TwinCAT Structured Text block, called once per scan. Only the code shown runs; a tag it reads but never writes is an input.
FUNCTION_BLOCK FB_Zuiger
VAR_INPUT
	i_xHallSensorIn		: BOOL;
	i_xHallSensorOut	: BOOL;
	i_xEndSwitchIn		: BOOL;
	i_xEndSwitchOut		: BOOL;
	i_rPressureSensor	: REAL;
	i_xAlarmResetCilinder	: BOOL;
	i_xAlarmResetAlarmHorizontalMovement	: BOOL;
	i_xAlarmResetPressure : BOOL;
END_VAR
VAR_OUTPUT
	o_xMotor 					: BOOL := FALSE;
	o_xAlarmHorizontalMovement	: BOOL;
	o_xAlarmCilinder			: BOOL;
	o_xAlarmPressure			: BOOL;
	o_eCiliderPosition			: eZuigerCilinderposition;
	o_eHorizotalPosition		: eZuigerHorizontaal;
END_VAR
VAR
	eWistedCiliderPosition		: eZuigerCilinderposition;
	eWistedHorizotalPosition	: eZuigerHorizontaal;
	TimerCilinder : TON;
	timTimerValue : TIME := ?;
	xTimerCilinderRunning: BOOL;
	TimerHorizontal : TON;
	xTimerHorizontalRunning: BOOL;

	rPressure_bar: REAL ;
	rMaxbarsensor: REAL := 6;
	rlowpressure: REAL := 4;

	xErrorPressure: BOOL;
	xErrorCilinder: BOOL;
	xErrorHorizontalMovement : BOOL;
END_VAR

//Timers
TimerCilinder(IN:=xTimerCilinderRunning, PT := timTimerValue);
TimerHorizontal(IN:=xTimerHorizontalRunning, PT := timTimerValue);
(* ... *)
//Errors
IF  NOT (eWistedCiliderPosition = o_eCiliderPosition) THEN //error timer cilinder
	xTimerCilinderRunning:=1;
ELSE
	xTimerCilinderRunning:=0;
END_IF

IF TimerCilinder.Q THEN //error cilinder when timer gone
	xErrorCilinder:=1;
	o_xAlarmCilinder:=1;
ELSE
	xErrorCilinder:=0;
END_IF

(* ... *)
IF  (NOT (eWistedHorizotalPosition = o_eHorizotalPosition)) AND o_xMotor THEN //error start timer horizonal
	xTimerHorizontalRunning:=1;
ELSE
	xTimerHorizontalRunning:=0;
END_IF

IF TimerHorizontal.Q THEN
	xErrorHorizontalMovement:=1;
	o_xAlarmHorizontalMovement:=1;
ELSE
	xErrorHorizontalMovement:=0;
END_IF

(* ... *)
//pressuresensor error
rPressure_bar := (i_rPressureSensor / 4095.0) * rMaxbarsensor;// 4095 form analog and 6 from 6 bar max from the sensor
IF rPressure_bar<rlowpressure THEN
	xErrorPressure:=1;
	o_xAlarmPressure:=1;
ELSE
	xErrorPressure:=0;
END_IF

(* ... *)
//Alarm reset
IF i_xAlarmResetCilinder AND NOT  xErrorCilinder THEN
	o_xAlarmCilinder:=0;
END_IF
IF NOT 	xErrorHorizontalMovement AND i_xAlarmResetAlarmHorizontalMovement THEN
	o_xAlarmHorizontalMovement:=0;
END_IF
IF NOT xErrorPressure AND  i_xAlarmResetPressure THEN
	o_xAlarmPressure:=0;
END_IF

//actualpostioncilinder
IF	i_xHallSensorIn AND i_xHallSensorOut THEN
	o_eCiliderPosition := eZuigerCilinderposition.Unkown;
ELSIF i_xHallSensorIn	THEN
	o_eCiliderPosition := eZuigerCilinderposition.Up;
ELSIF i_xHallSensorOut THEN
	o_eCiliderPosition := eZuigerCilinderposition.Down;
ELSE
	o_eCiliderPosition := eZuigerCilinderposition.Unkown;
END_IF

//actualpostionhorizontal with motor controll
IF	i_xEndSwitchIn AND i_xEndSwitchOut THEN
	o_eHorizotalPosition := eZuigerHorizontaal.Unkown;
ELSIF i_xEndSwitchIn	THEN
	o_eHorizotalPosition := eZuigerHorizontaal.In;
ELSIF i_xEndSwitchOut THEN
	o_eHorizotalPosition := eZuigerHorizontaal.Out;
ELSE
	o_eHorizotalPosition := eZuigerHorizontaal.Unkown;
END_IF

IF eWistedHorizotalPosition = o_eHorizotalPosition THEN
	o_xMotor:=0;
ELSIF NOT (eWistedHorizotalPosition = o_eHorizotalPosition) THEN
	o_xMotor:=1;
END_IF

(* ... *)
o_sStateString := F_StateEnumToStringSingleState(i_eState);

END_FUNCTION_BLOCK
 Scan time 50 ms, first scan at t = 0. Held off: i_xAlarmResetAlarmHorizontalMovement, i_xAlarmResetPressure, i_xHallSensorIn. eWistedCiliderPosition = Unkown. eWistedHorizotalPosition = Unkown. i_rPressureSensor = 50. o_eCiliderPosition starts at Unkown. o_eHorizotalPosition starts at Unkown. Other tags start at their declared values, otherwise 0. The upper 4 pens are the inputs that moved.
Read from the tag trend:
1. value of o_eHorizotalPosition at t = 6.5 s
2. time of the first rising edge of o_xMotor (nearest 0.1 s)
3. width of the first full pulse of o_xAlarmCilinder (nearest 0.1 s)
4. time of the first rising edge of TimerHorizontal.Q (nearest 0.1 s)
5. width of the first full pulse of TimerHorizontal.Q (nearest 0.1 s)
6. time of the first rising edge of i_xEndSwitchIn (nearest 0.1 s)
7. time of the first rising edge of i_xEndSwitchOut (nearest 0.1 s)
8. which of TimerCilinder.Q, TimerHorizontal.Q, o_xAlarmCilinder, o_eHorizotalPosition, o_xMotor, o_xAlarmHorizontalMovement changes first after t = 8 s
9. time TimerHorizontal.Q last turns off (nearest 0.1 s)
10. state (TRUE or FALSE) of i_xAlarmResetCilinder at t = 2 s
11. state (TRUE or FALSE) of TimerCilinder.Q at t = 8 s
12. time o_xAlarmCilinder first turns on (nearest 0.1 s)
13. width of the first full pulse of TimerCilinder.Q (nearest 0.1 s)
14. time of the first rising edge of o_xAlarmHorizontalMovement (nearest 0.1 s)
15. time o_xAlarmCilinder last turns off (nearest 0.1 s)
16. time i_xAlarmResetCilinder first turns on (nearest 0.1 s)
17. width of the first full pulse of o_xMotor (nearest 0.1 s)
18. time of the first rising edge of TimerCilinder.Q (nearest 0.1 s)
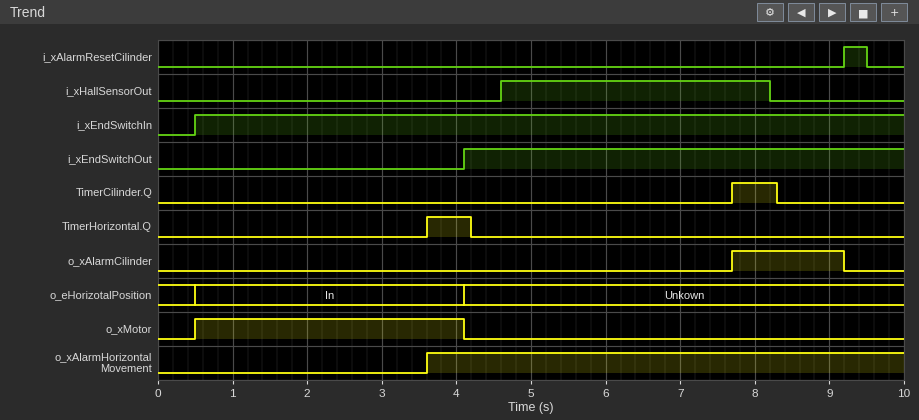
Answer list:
Unkown
0.5 s
1.5 s
3.6 s
0.6 s
0.5 s
4.1 s
TimerCilinder.Q
4.2 s
FALSE
TRUE
7.7 s
0.6 s
3.6 s
9.2 s
9.2 s
3.6 s
7.7 s
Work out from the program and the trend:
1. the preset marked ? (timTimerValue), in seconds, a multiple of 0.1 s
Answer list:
3.0 s
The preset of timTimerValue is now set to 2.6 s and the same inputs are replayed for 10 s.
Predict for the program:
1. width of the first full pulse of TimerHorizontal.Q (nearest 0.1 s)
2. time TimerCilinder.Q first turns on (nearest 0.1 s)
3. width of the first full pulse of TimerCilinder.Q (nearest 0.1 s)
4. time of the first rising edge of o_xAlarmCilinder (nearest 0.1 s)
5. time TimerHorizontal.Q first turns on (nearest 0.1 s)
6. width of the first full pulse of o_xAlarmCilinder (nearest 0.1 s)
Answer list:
1.0 s
7.3 s
1.0 s
7.3 s
3.2 s
1.9 s
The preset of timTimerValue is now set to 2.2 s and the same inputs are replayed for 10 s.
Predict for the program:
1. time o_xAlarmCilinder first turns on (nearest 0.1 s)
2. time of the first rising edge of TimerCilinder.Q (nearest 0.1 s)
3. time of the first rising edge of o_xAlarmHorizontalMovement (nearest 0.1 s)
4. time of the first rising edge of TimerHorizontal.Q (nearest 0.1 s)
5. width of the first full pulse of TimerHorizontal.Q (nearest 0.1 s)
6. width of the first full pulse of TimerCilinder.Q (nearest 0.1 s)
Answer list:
6.9 s
6.9 s
2.8 s
2.8 s
1.4 s
1.4 s
